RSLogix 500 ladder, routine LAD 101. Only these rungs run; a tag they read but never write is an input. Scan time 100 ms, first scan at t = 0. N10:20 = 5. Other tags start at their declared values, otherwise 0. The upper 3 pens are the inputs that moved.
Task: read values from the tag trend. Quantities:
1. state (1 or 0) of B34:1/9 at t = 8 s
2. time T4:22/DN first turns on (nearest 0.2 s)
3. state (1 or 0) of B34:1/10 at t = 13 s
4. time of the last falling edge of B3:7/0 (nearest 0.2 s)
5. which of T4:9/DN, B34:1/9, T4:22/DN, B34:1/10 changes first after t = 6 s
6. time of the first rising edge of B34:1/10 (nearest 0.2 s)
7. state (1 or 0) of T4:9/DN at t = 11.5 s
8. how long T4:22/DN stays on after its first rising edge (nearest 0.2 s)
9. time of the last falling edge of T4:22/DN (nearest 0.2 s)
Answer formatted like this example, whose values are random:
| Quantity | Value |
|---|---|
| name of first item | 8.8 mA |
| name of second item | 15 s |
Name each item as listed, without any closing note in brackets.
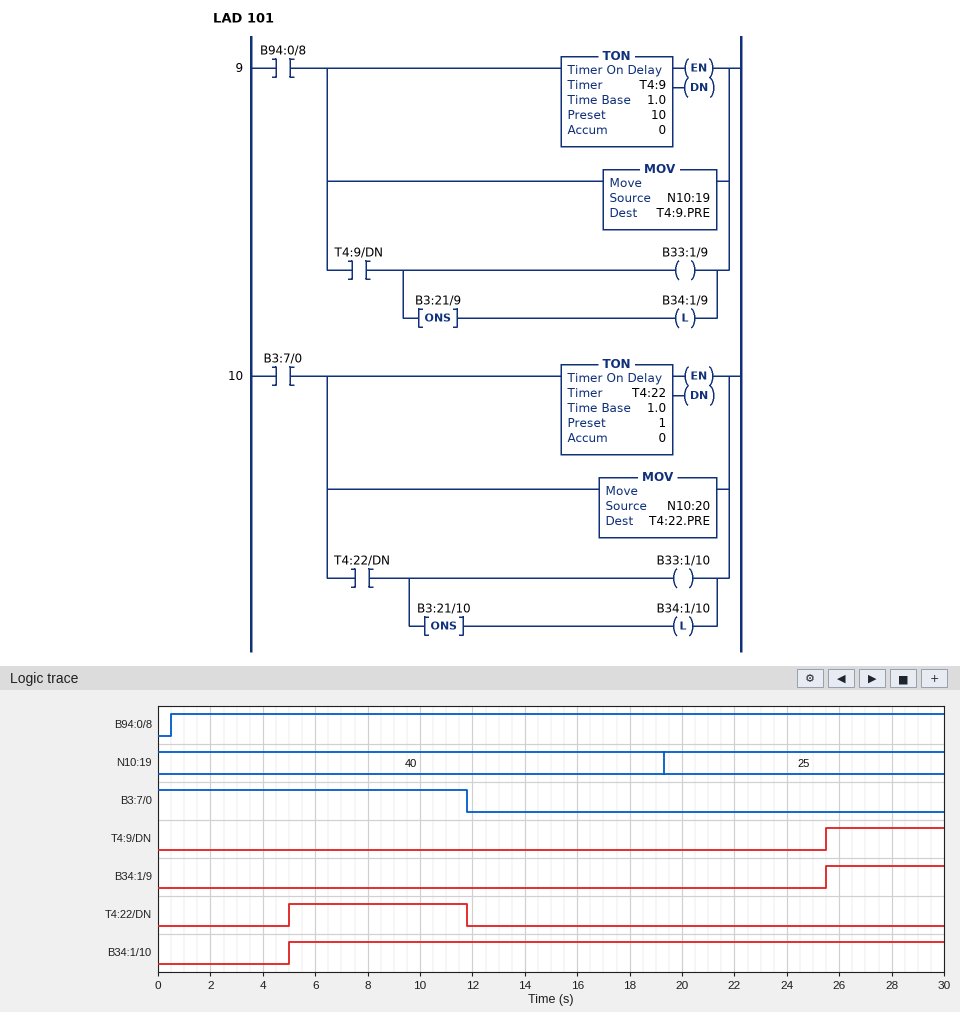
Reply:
| Quantity | Value |
|---|---|
| state (1 or 0) of B34:1/9 at t = 8 s | 0 |
| time T4:22/DN first turns on | 5.0 s |
| state (1 or 0) of B34:1/10 at t = 13 s | 1 |
| time of the last falling edge of B3:7/0 | 11.8 s |
| which of T4:9/DN, B34:1/9, T4:22/DN, B34:1/10 changes first after t = 6 s | T4:22/DN |
| time of the first rising edge of B34:1/10 | 5.0 s |
| state (1 or 0) of T4:9/DN at t = 11.5 s | 0 |
| how long T4:22/DN stays on after its first rising edge | 6.8 s |
| time of the last falling edge of T4:22/DN | 11.8 s |
